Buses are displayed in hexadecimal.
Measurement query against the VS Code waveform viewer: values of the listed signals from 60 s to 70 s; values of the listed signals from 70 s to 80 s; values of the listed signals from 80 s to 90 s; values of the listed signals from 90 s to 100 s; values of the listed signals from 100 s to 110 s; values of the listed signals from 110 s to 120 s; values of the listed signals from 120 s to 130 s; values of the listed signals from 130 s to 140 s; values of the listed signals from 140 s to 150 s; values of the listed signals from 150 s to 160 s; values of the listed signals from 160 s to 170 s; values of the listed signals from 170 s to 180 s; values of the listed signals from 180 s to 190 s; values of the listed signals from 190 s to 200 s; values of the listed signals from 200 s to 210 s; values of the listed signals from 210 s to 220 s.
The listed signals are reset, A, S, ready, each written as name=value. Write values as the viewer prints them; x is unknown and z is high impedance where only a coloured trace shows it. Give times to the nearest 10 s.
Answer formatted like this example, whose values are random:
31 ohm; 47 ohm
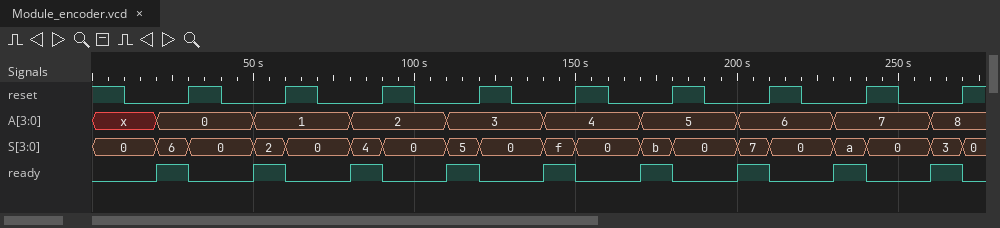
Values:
reset=1, A=1, S=0, ready=0; reset=0, A=1, S=0, ready=0; reset=0, A=2, S=4, ready=1; reset=1, A=2, S=0, ready=0; reset=0, A=2, S=0, ready=0; reset=0, A=3, S=5, ready=1; reset=1, A=3, S=0, ready=0; reset=0, A=3, S=0, ready=0; reset=0, A=4, S=f, ready=1; reset=1, A=4, S=0, ready=0; reset=0, A=4, S=0, ready=0; reset=0, A=5, S=b, ready=1; reset=1, A=5, S=0, ready=0; reset=0, A=5, S=0, ready=0; reset=0, A=6, S=7, ready=1; reset=1, A=6, S=0, ready=0
